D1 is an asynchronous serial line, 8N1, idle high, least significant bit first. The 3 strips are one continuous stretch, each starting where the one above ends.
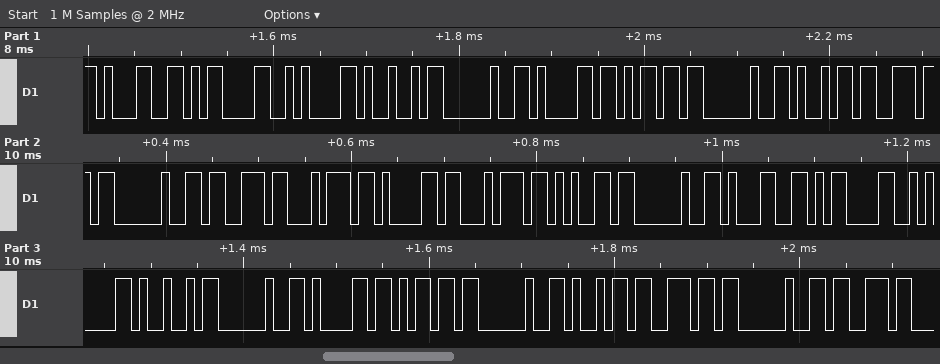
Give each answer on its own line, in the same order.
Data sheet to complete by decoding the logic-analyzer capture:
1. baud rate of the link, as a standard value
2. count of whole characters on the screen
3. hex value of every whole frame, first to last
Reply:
115200 baud
29
31 0D 0A 49 20 61 6D 20 69 6E 20 73 74 61 74 65 20 31 0D 0A 49 20 61 6D 20 69 6E 20 73
